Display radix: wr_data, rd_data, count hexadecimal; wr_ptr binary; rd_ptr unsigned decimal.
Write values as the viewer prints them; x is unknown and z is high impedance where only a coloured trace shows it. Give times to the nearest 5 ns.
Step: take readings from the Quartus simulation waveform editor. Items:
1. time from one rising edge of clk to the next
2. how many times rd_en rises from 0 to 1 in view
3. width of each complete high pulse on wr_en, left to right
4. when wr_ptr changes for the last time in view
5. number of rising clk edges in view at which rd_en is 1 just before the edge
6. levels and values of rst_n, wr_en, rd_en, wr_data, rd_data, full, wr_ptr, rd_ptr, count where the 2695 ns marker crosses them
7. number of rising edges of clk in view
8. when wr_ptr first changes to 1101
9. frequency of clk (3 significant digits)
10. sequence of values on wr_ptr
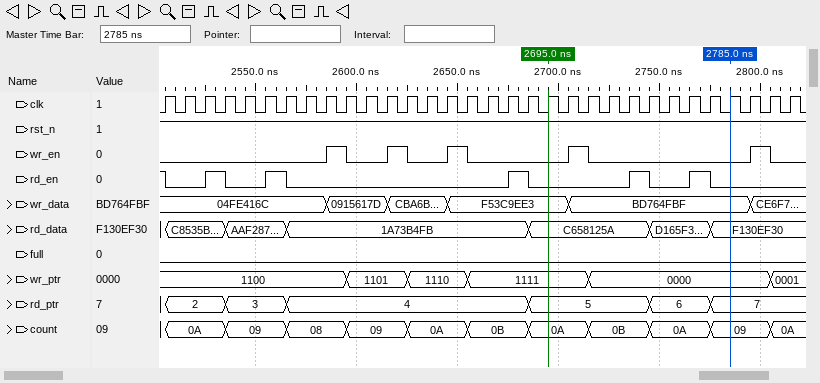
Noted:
10 ns
5
10 ns, 10 ns, 10 ns, 10 ns, 10 ns
2805 ns
6
rst_n=1, wr_en=0, rd_en=0, wr_data=F53C9EE3, rd_data=C658125A, full=0, wr_ptr=1111, rd_ptr=5, count=0A
32
2595 ns
100 MHz
1100, 1101, 1110, 1111, 0000, 0001
